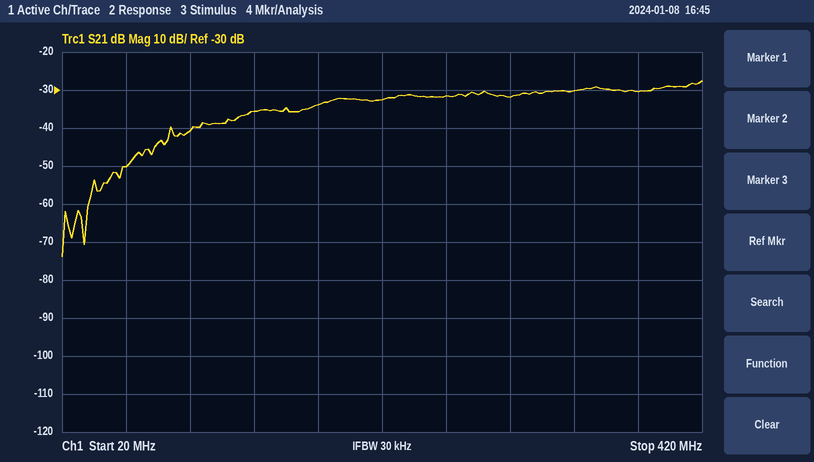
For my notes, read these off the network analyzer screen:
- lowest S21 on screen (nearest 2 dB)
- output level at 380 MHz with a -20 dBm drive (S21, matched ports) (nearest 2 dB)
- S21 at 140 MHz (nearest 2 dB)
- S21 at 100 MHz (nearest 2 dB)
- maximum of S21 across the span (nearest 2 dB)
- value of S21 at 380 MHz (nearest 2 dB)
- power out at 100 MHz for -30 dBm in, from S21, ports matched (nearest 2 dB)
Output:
-74 dB
-50 dBm
-36 dB
-40 dB
-28 dB
-30 dB
-70 dBm
